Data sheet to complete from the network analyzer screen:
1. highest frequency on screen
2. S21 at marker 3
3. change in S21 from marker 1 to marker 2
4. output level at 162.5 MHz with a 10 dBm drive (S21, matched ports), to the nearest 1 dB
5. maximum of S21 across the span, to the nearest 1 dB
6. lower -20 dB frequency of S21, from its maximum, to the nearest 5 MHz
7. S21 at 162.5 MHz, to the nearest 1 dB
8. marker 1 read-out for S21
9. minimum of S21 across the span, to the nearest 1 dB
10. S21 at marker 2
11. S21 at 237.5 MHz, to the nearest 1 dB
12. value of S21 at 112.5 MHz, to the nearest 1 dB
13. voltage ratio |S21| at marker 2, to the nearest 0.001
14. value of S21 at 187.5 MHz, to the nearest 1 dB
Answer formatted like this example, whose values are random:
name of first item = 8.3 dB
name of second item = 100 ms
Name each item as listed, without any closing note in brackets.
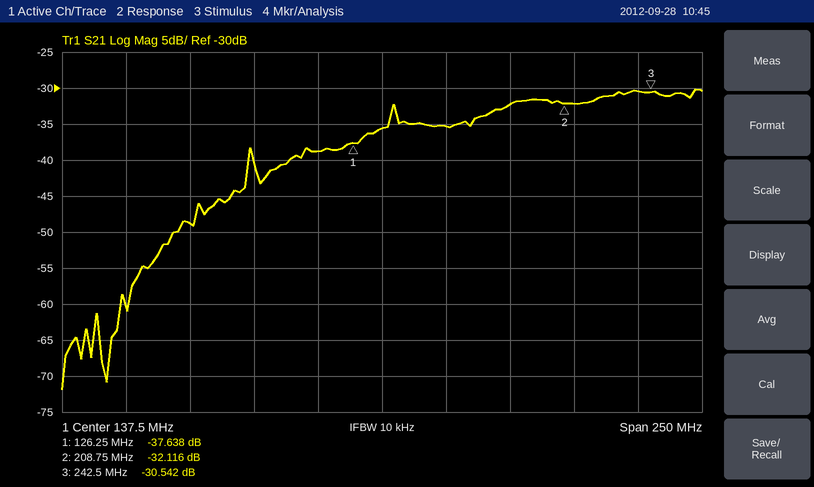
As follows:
highest frequency on screen = 262.5 MHz
S21 at marker 3 = -30.542 dB
change in S21 from marker 1 to marker 2 = 5.522 dB
output level at 162.5 MHz with a 10 dBm drive (S21, matched ports), to the nearest 1 dB = -25 dBm
maximum of S21 across the span, to the nearest 1 dB = -30 dB
lower -20 dB frequency of S21, from its maximum, to the nearest 5 MHz = 55 MHz
S21 at 162.5 MHz, to the nearest 1 dB = -35 dB
marker 1 read-out for S21 = -37.638 dB
minimum of S21 across the span, to the nearest 1 dB = -72 dB
S21 at marker 2 = -32.116 dB
S21 at 237.5 MHz, to the nearest 1 dB = -30 dB
value of S21 at 112.5 MHz, to the nearest 1 dB = -39 dB
voltage ratio |S21| at marker 2, to the nearest 0.001 = 0.025
value of S21 at 187.5 MHz, to the nearest 1 dB = -32 dB
